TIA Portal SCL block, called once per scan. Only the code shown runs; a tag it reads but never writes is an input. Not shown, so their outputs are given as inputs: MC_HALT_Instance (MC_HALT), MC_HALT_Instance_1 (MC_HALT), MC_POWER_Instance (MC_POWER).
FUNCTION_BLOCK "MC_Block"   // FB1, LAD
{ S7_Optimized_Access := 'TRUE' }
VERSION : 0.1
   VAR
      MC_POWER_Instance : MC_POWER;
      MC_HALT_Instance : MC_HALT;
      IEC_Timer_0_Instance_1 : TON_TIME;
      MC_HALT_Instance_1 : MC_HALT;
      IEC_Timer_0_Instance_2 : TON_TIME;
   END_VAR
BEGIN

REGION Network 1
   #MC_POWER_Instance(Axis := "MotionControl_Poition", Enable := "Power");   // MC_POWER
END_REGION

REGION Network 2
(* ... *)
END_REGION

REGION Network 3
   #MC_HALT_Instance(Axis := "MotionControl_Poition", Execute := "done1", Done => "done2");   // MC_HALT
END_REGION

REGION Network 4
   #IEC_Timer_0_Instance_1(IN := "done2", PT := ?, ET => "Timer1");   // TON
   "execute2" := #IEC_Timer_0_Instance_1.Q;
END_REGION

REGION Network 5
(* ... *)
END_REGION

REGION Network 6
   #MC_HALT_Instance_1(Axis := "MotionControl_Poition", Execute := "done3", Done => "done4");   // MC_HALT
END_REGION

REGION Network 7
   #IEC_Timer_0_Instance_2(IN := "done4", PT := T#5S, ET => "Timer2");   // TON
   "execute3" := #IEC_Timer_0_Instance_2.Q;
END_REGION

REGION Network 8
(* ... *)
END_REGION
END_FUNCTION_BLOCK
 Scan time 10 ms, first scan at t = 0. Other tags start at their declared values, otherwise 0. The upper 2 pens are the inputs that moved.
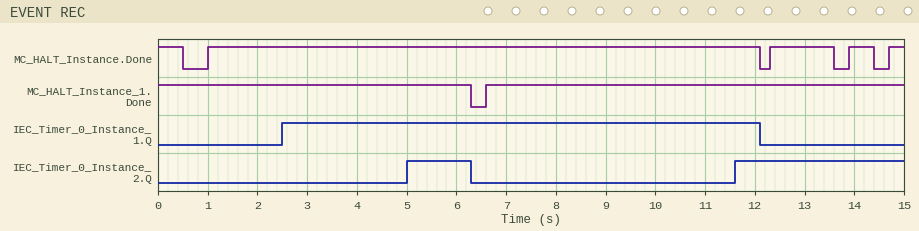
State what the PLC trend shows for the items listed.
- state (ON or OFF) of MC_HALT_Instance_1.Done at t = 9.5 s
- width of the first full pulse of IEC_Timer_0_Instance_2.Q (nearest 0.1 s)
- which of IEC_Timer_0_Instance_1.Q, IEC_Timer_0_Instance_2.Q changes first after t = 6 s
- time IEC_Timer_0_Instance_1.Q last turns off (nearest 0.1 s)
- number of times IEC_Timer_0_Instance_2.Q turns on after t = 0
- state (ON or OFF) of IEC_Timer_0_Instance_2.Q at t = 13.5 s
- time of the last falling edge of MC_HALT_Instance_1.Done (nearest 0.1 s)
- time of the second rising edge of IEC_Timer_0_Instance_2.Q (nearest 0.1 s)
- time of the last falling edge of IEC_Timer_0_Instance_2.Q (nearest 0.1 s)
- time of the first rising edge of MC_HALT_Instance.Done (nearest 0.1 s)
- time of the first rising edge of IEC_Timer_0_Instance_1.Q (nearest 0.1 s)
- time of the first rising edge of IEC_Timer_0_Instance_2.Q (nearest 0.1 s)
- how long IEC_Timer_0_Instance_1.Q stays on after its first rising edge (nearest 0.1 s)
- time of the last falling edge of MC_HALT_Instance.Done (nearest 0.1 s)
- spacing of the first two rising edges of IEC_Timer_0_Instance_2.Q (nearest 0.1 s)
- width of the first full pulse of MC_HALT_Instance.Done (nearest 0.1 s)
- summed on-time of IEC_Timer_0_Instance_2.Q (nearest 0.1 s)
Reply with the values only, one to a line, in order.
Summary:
ON
1.3 s
IEC_Timer_0_Instance_2.Q
12.1 s
2
ON
6.3 s
11.6 s
6.3 s
1.0 s
2.5 s
5.0 s
9.6 s
14.4 s
6.6 s
11.1 s
4.7 s
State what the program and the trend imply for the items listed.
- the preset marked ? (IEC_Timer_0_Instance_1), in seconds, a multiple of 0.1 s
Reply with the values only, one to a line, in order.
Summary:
1.5 s
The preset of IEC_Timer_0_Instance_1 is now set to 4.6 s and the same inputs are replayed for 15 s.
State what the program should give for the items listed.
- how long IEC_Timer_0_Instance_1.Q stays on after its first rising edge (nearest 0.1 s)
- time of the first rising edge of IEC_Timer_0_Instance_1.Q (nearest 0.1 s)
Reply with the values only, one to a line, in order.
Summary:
6.5 s
5.6 s
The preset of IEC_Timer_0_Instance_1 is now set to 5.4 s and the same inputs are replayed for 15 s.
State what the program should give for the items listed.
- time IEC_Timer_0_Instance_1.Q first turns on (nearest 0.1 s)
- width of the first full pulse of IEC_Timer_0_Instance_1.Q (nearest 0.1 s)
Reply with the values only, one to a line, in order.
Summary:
6.4 s
5.7 s
